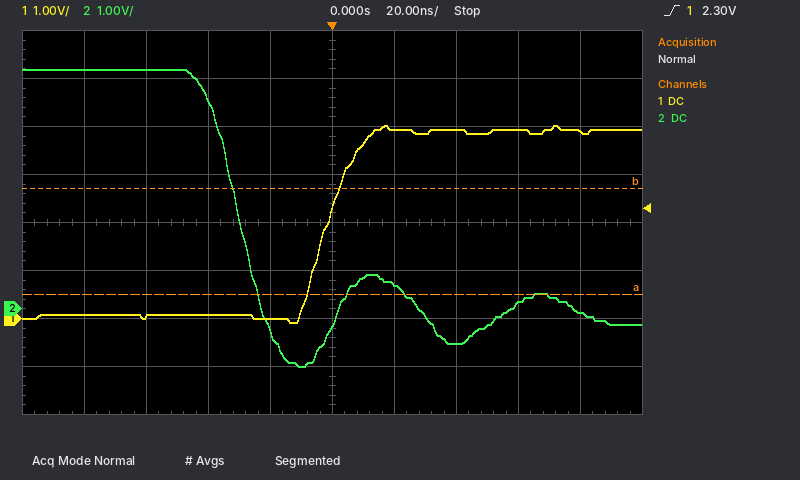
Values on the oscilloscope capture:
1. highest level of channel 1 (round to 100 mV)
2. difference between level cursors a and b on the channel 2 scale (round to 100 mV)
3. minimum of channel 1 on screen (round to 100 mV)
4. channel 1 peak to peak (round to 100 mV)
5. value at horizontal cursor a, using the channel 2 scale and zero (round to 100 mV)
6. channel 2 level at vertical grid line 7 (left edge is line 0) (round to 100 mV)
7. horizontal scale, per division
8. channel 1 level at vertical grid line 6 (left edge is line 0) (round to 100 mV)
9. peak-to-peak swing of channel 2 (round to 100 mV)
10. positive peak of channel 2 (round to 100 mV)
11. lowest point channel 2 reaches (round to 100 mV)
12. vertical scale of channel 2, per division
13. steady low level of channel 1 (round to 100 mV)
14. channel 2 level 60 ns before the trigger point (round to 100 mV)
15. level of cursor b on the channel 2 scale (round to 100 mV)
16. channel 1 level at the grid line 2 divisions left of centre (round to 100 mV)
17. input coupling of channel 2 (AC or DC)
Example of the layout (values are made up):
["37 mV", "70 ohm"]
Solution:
["4.0 V", "2.2 V", "-100 mV", "4.1 V", "300 mV", "-700 mV", "20 ns", "3.9 V", "6.2 V", "5.0 V", "-1.2 V", "1 V", "100 mV", "5.0 V", "2.5 V", "100 mV", "DC"]
